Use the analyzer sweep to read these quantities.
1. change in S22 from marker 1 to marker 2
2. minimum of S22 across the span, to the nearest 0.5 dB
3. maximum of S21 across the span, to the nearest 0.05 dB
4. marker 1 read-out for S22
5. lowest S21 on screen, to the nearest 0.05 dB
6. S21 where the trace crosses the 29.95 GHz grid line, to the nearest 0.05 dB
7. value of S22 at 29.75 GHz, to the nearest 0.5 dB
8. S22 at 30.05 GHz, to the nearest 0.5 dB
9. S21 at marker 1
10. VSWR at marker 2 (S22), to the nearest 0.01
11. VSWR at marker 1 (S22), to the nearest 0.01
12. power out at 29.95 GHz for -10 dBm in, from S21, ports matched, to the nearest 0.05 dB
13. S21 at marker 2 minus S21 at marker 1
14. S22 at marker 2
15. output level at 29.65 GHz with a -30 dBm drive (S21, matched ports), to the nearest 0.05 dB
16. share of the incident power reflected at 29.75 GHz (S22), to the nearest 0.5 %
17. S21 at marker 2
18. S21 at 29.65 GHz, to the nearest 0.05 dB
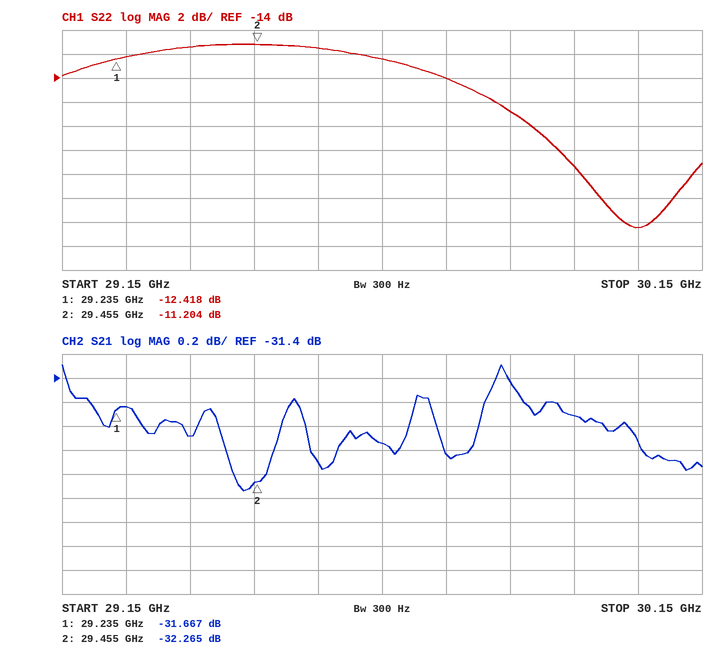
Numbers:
1.214 dB
-26.5 dB
-31.30 dB
-12.418 dB
-32.35 dB
-31.70 dB
-14.0 dB
-26.5 dB
-31.667 dB
1.76
1.63
-41.70 dBm
-0.598 dB
-11.204 dB
-61.95 dBm
4.0 %
-32.265 dB
-31.95 dB
